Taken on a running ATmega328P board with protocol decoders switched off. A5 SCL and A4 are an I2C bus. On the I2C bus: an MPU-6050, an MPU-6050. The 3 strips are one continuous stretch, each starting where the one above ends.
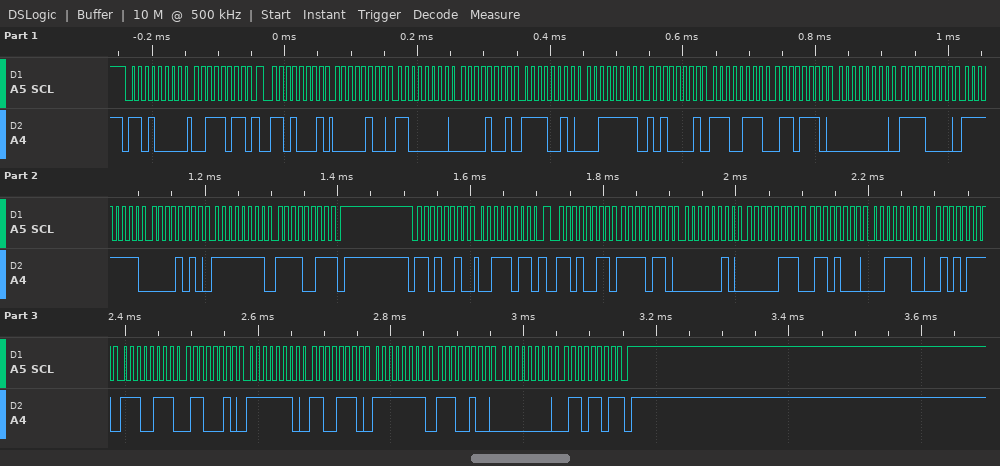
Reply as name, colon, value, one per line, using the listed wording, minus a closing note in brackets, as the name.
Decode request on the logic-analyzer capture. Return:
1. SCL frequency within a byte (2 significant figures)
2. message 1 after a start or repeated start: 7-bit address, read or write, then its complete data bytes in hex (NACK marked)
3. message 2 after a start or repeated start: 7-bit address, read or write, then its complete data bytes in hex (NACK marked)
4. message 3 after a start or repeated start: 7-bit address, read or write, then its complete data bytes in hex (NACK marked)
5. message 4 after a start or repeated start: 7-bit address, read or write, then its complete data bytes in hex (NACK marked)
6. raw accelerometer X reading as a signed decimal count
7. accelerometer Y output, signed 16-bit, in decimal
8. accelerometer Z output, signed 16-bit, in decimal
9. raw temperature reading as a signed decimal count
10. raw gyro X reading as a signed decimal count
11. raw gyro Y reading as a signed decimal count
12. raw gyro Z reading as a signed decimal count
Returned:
SCL frequency within a byte: 100 kHz
message 1 after a start or repeated start: 7-bit address, read or write, then its complete data bytes in hex: 0x68 write: 3B
message 2 after a start or repeated start: 7-bit address, read or write, then its complete data bytes in hex: 0x68 read: 04 C0 09 F2 3F A1 E7 6E 00 F0 FF 0A FF F3 NACK
message 3 after a start or repeated start: 7-bit address, read or write, then its complete data bytes in hex: 0x69 write: 3B
message 4 after a start or repeated start: 7-bit address, read or write, then its complete data bytes in hex: 0x69 read: F6 02 07 68 3C 57 E7 62 FE CE FF E4 00 6D NACK
raw accelerometer X reading as a signed decimal count: 1216
accelerometer Y output, signed 16-bit, in decimal: 2546
accelerometer Z output, signed 16-bit, in decimal: 16289
raw temperature reading as a signed decimal count: -6290
raw gyro X reading as a signed decimal count: 240
raw gyro Y reading as a signed decimal count: -246
raw gyro Z reading as a signed decimal count: -13
